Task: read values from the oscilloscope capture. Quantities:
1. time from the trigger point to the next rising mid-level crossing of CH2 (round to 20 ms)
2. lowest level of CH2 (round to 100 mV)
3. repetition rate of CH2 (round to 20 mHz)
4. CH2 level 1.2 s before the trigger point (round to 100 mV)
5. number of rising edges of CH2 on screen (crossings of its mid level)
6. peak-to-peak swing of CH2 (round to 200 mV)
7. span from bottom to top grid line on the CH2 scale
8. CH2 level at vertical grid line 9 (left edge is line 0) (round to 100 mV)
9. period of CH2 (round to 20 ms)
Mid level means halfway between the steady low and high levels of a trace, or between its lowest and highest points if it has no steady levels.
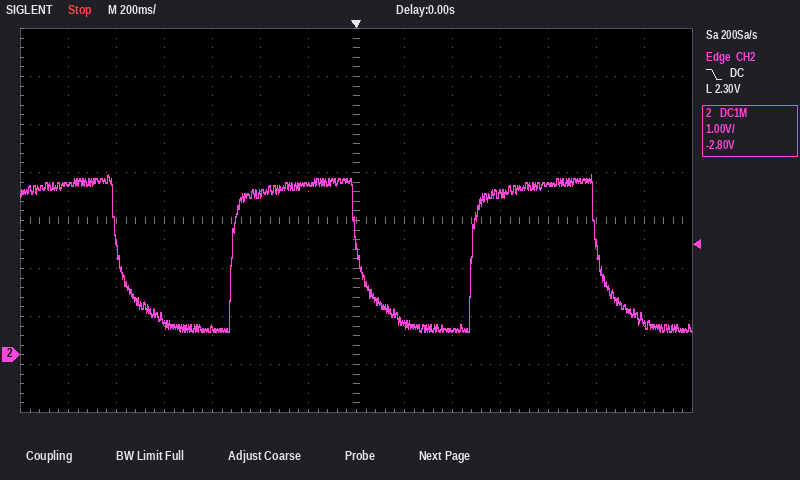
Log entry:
480 ms
500 mV
1.00 Hz
3.6 V
2
3.2 V
8 V
500 mV
1.00 s
